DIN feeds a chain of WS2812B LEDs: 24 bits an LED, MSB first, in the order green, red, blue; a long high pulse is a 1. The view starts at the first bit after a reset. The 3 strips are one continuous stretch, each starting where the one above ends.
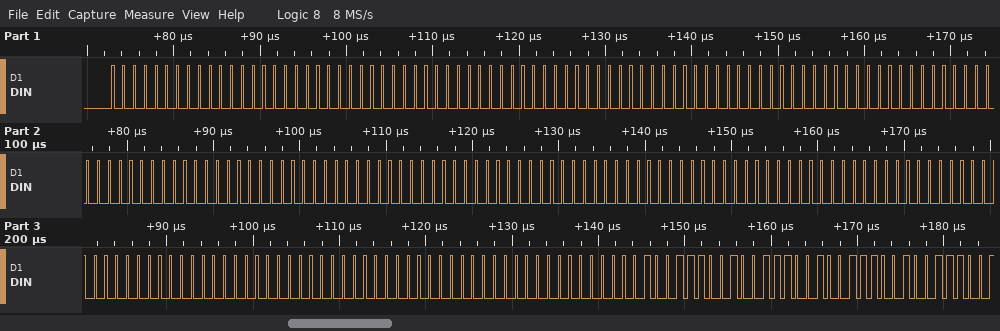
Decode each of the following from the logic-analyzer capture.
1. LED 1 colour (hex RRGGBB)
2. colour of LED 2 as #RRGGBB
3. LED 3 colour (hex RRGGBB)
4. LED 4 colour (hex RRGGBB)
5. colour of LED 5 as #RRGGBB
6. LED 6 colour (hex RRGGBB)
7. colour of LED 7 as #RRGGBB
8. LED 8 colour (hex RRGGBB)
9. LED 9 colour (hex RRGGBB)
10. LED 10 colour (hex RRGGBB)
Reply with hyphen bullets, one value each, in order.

- #000000
- #000000
- #000000
- #000000
- #000000
- #000000
- #000000
- #000000
- #000000
- #272727
